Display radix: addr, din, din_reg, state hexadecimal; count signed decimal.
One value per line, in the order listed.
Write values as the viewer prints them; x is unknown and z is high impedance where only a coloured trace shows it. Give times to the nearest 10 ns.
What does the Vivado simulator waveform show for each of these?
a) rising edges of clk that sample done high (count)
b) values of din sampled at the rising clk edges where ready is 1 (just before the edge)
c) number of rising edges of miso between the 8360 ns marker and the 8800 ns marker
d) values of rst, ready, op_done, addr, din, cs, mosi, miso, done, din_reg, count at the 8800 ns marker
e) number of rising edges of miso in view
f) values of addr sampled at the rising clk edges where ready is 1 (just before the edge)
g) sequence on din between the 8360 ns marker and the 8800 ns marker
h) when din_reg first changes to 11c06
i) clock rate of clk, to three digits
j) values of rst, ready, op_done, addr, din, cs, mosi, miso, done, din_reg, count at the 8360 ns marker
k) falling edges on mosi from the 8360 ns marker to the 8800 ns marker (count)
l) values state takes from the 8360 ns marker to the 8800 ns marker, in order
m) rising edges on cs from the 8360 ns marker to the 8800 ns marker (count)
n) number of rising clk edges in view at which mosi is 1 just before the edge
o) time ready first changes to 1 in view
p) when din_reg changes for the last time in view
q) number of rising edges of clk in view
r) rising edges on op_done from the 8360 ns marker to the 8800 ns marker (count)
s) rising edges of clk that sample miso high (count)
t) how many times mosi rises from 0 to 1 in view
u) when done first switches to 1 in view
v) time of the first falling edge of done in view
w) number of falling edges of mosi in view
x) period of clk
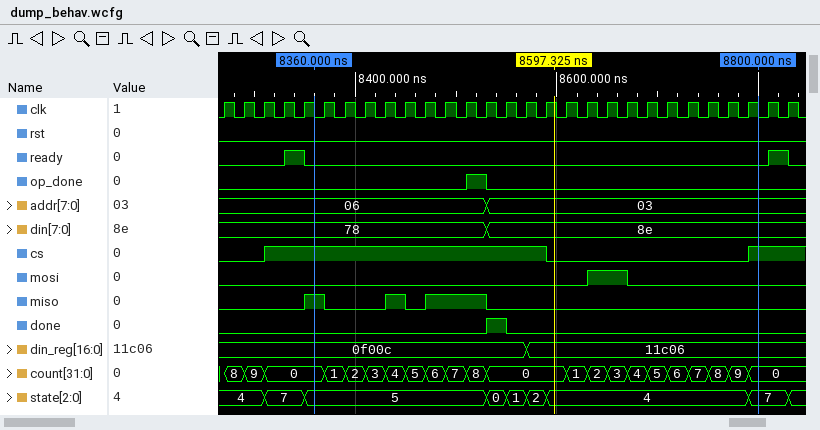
1
78, 8e
2
rst=0, ready=0, op_done=0, addr=03, din=8e, cs=1, mosi=0, miso=0, done=0, din_reg=11c06, count=0
3
06, 03
78, 8e
8570 ns
50.0 MHz
rst=0, ready=0, op_done=0, addr=06, din=78, cs=1, mosi=0, miso=1, done=0, din_reg=0f00c, count=0
1
5, 0, 1, 2, 4, 7
1
2
8330 ns
8570 ns
29
1
5
1
8530 ns
8550 ns
1
20 ns
